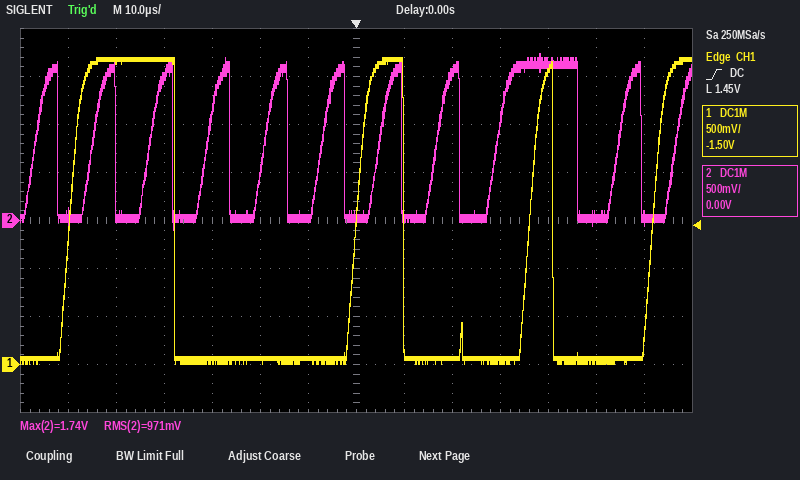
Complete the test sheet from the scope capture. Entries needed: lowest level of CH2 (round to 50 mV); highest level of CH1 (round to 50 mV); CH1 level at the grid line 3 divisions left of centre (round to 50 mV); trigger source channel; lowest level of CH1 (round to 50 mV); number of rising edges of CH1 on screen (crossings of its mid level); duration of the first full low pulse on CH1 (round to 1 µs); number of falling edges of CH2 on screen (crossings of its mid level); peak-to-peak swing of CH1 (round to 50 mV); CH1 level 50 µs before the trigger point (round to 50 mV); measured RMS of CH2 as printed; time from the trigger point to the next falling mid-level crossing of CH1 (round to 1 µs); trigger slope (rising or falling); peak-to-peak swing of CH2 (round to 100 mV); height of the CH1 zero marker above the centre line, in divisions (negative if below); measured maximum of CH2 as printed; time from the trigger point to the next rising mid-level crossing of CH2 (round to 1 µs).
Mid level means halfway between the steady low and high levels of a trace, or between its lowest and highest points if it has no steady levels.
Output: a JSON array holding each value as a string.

["-100 mV", "3.20 V", "50 mV", "CH1", "0 mV", "4", "38 µs", "10", "3.20 V", "3.15 V", "971 mV", "10 µs", "rising", "1.80 V", "-3.0 div", "1.74 V", "5 µs"]
